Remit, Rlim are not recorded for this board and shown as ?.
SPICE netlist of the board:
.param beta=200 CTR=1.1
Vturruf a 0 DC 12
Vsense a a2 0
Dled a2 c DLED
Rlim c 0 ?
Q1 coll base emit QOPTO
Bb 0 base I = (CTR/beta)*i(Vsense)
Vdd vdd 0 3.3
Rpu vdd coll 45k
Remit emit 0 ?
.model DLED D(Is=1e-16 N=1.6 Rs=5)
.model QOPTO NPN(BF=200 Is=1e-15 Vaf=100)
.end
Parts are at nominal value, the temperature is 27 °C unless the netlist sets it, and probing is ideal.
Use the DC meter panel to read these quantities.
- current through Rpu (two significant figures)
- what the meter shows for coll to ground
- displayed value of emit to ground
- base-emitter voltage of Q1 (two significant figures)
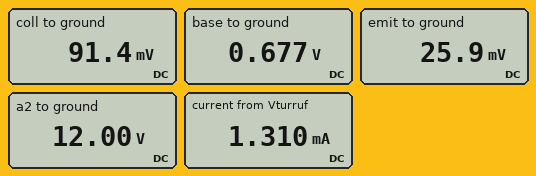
71 µA
91.4 mV
25.9 mV
650 mV
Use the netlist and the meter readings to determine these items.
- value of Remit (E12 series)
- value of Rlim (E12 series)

330 Ω
8.2 kΩ
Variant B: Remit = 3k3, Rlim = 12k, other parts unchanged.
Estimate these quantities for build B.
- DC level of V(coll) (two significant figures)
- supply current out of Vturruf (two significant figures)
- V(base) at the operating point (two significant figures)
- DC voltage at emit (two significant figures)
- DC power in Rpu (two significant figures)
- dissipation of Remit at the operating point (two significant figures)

310 mV
900 µA
880 mV
240 mV
200 µW
17 µW
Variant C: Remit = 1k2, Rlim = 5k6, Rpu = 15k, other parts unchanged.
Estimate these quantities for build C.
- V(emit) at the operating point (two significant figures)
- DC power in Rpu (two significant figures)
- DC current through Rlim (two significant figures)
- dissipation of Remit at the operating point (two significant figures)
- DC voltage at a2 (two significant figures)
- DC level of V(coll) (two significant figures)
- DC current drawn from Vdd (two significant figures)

250 mV
590 µW
1.9 mA
52 µW
12 V
330 mV
200 µA
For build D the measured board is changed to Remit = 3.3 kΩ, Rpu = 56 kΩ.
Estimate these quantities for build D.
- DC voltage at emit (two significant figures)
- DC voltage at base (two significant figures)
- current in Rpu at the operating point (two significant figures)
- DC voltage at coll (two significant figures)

200 mV
850 mV
54 µA
260 mV
